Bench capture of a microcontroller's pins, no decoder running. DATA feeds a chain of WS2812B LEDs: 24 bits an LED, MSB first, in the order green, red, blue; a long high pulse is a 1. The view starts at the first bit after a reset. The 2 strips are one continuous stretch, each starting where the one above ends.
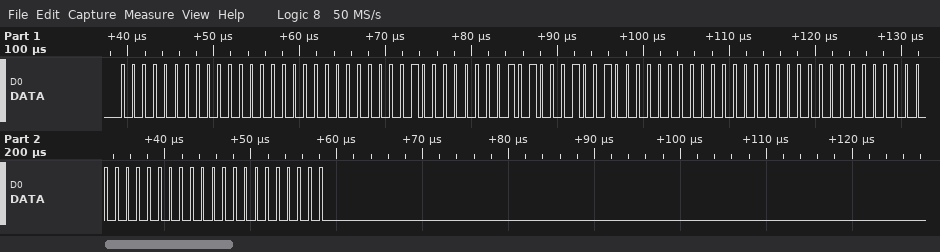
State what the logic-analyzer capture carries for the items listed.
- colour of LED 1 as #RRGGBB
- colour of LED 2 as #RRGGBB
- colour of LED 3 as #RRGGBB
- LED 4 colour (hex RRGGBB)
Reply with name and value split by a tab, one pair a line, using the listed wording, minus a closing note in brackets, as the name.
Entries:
colour of LED 1 as #RRGGBB	#000000
colour of LED 2 as #RRGGBB	#0A1024
colour of LED 3 as #RRGGBB	#000000
LED 4 colour	#000000
